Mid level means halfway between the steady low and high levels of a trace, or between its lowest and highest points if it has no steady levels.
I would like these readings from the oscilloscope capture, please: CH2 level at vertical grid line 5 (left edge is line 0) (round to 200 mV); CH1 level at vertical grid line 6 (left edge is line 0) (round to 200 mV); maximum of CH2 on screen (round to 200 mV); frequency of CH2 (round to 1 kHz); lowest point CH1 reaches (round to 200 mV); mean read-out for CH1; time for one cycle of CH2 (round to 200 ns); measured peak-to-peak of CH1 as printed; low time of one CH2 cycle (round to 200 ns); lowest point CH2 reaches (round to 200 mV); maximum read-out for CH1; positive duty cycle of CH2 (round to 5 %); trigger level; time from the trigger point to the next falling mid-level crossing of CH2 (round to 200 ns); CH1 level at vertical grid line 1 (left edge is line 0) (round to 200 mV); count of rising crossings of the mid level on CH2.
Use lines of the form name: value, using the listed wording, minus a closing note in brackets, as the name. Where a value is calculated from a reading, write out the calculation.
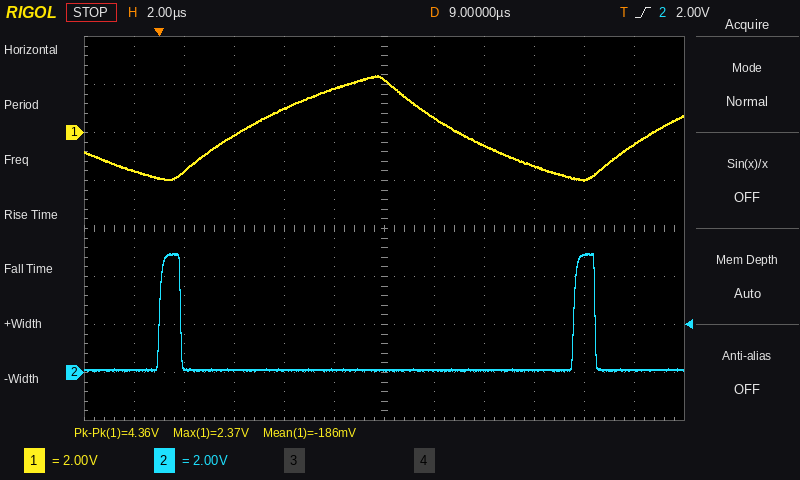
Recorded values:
CH2 level at vertical grid line 5 (left edge is line 0): 200 mV
CH1 level at vertical grid line 6 (left edge is line 0): 2.2 V
maximum of CH2 on screen: 5.0 V
frequency of CH2: 1 / 16.6 µs ≈ 60 kHz
lowest point CH1 reaches: -2.0 V
mean read-out for CH1: -186 mV
time for one cycle of CH2: 16.6 µs
measured peak-to-peak of CH1 as printed: 4.36 V
low time of one CH2 cycle: 15.8 µs
lowest point CH2 reaches: 0.0 V
maximum read-out for CH1: 2.37 V
positive duty cycle of CH2: 5 %
trigger level: 2.00 V
time from the trigger point to the next falling mid-level crossing of CH2: 800 ns
CH1 level at vertical grid line 1 (left edge is line 0): -1.6 V
count of rising crossings of the mid level on CH2: 2
